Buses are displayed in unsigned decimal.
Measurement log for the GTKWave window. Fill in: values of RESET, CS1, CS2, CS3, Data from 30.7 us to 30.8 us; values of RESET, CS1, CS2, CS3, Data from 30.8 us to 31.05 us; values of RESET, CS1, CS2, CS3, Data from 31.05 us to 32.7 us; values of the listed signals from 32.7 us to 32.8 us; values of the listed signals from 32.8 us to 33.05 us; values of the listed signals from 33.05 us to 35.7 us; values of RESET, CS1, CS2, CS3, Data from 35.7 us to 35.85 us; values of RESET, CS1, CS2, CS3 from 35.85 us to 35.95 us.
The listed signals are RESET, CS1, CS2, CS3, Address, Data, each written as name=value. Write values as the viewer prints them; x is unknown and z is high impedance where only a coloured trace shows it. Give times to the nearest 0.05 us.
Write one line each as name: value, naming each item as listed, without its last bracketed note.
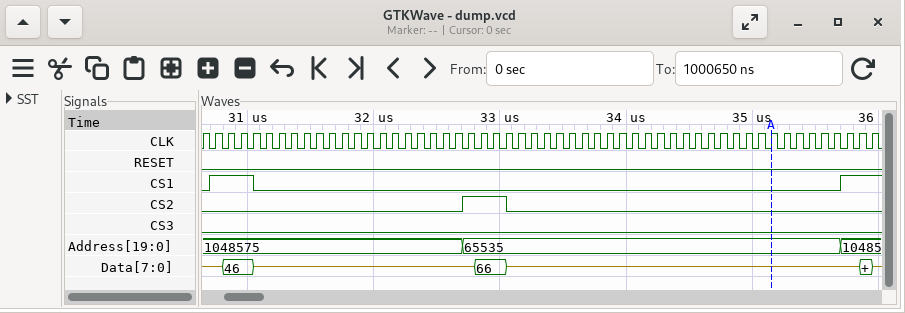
values of RESET, CS1, CS2, CS3, Data from 30.7 us to 30.8 us: RESET=0, CS1=1, CS2=0, CS3=0, Data=z
values of RESET, CS1, CS2, CS3, Data from 30.8 us to 31.05 us: RESET=0, CS1=1, CS2=0, CS3=0, Data=46
values of RESET, CS1, CS2, CS3, Data from 31.05 us to 32.7 us: RESET=0, CS1=0, CS2=0, CS3=0, Data=z
values of the listed signals from 32.7 us to 32.8 us: RESET=0, CS1=0, CS2=1, CS3=0, Address=65535, Data=z
values of the listed signals from 32.8 us to 33.05 us: RESET=0, CS1=0, CS2=1, CS3=0, Address=65535, Data=66
values of the listed signals from 33.05 us to 35.7 us: RESET=0, CS1=0, CS2=0, CS3=0, Address=65535, Data=z
values of RESET, CS1, CS2, CS3, Data from 35.7 us to 35.85 us: RESET=0, CS1=1, CS2=0, CS3=0, Data=z
values of RESET, CS1, CS2, CS3 from 35.85 us to 35.95 us: RESET=0, CS1=1, CS2=0, CS3=0
